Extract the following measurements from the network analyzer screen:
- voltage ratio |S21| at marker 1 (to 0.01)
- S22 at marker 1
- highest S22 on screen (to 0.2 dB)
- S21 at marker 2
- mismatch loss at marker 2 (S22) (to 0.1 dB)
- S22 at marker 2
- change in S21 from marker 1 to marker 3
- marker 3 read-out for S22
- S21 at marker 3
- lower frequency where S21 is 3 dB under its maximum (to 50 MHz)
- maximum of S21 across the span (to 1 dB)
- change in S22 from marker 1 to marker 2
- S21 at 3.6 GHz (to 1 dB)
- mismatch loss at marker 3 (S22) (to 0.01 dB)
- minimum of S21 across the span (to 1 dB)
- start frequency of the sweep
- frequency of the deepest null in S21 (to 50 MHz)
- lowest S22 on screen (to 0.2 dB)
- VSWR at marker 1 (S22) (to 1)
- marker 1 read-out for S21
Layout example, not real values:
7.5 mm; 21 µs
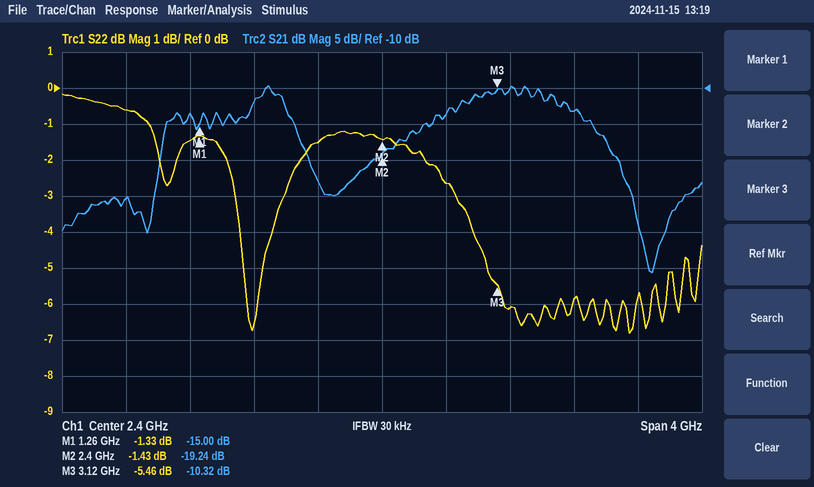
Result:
0.18; -1.33 dB; -0.2 dB; -19.24 dB; 5.5 dB; -1.43 dB; 4.68 dB; -5.46 dB; -10.32 dB; 1.60 GHz; -10 dB; -0.10 dB; -13 dB; 1.45 dB; -36 dB; 400 MHz; 4.10 GHz; -6.8 dB; 13; -15.00 dB
